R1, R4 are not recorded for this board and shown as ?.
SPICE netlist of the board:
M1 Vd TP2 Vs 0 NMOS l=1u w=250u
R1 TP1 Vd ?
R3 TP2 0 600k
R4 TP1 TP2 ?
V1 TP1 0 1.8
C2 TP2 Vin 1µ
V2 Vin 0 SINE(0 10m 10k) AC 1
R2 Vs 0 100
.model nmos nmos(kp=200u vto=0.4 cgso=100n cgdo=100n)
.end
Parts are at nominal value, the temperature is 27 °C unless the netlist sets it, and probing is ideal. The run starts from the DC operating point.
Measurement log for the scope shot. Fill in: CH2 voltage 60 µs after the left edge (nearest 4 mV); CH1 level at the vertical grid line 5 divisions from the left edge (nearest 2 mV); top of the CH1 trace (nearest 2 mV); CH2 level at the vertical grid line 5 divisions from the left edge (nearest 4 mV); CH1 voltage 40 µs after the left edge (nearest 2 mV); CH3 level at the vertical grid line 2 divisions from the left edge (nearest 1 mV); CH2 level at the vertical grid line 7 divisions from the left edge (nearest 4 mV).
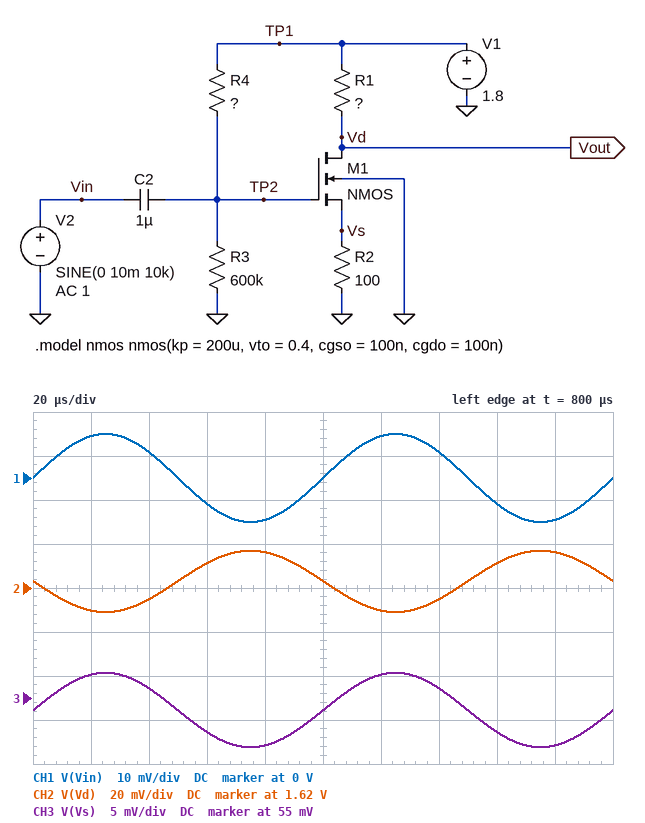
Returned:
1.632 V
0 V
10 mV
1.624 V
6 mV
56 mV
1.616 V
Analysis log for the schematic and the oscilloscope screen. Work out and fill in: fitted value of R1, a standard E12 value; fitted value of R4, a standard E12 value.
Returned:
330 Ω
1.2 MΩ
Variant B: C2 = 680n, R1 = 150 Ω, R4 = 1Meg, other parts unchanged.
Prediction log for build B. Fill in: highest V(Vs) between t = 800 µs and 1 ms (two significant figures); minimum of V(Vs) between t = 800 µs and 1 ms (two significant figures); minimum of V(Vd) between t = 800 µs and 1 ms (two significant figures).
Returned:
93 mV
83 mV
1.7 V
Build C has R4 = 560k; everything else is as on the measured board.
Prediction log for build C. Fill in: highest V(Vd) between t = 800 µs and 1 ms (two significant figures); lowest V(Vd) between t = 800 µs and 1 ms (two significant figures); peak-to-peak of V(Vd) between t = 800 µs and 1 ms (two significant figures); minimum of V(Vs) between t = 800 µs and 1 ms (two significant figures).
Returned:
1.1 V
1.0 V
40 mV
220 mV
